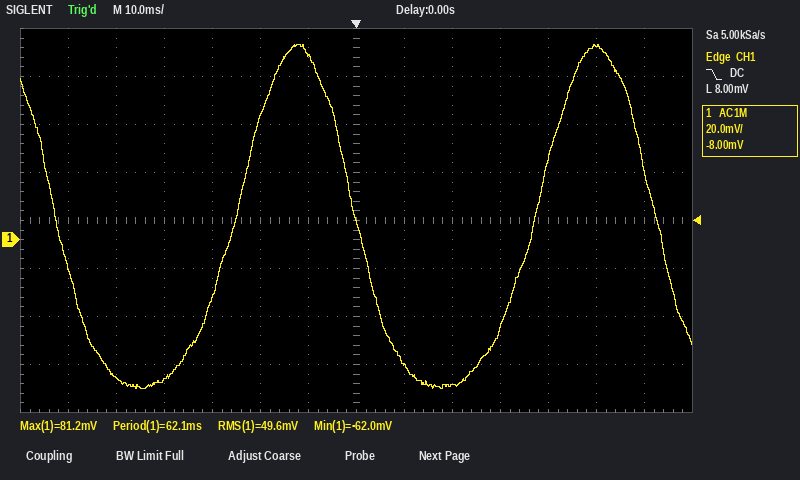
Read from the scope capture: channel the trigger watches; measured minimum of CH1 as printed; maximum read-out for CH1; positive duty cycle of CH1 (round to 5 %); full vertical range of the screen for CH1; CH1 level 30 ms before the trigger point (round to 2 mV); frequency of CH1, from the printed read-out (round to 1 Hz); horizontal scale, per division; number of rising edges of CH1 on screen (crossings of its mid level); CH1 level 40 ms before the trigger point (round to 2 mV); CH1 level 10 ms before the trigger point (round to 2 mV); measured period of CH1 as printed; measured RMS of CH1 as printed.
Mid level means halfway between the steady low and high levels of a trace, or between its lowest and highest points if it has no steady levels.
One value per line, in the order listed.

CH1
-62.0 mV
81.2 mV
40 %
160 mV
-24 mV
16 Hz
10 ms
2
-58 mV
78 mV
62.1 ms
49.6 mV
